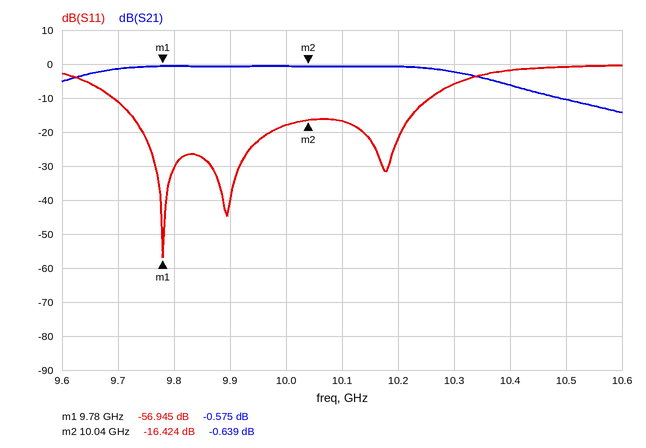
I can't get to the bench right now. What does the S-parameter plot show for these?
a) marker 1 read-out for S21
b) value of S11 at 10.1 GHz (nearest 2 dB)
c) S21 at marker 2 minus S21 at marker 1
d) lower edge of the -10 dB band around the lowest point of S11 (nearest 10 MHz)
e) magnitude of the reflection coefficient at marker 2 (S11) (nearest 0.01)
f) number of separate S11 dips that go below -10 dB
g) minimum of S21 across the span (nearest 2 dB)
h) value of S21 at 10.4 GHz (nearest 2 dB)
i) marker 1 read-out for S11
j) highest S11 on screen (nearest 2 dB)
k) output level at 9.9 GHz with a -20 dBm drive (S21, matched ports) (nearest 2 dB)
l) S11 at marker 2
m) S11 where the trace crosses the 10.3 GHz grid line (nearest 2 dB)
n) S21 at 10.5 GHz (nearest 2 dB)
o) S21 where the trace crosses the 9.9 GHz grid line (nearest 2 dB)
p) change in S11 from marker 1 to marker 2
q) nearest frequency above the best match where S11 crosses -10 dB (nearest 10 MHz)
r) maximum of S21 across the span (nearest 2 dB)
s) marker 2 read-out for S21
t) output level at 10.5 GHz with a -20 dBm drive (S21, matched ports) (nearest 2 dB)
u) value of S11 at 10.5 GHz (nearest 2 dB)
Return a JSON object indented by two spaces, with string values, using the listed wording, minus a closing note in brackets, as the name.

{
  "marker 1 read-out for S21": "-0.575 dB",
  "value of S11 at 10.1 GHz": "-16 dB",
  "S21 at marker 2 minus S21 at marker 1": "-0.064 dB",
  "lower edge of the -10 dB band around the lowest point of S11": "9.69 GHz",
  "magnitude of the reflection coefficient at marker 2 (S11)": "0.15",
  "number of separate S11 dips that go below -10 dB": "3",
  "minimum of S21 across the span": "-14 dB",
  "value of S21 at 10.4 GHz": "-6 dB",
  "marker 1 read-out for S11": "-56.945 dB",
  "highest S11 on screen": "0 dB",
  "output level at 9.9 GHz with a -20 dBm drive (S21, matched ports)": "-20 dBm",
  "S11 at marker 2": "-16.424 dB",
  "S11 where the trace crosses the 10.3 GHz grid line": "-6 dB",
  "S21 at 10.5 GHz": "-10 dB",
  "S21 where the trace crosses the 9.9 GHz grid line": "0 dB",
  "change in S11 from marker 1 to marker 2": "40.521 dB",
  "nearest frequency above the best match where S11 crosses -10 dB": "10.26 GHz",
  "maximum of S21 across the span": "0 dB",
  "marker 2 read-out for S21": "-0.639 dB",
  "output level at 10.5 GHz with a -20 dBm drive (S21, matched ports)": "-30 dBm",
  "value of S11 at 10.5 GHz": "0 dB"
}
